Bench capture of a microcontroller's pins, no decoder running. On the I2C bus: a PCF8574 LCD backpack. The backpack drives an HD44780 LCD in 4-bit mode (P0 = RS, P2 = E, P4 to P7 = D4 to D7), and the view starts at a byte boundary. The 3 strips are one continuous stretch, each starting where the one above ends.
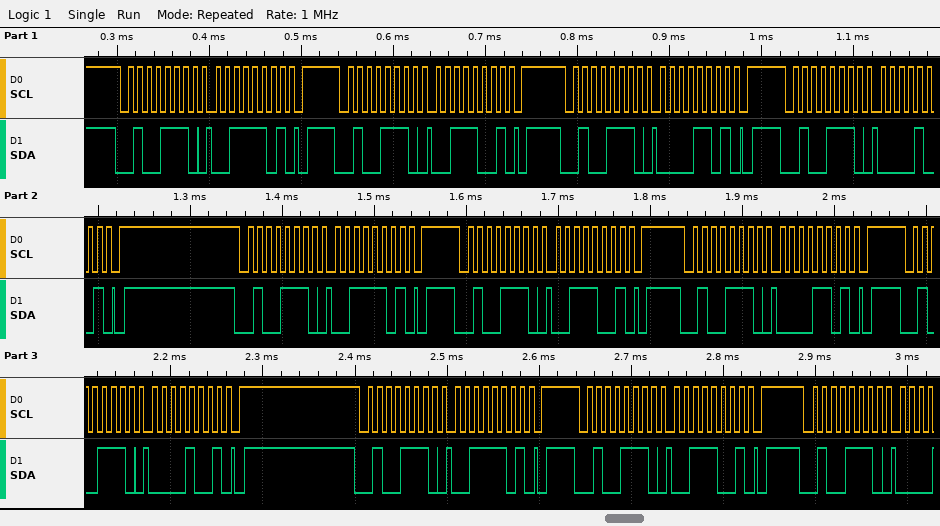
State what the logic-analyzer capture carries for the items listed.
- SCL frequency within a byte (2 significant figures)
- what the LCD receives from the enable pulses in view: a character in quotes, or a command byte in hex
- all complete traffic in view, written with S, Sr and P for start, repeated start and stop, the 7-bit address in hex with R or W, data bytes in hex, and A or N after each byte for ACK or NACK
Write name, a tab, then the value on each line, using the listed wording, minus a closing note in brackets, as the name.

SCL frequency within a byte	100 kHz
what the LCD receives from the enable pulses in view: a character in quotes, or a command byte in hex	'0' '0'
all complete traffic in view, written with S, Sr and P for start, repeated start and stop, the 7-bit address in hex with R or W, data bytes in hex, and A or N after each byte for ACK or NACK	S 27W A 3D A P S 27W A 39 A P S 27W A 0D A P S 27W A 09 A P S 27W A 3D A P S 27W A 39 A P S 27W A 0D A P S 27W A 09 A P S 27W A 3D A P S 27W A 39 A P S 27W A
